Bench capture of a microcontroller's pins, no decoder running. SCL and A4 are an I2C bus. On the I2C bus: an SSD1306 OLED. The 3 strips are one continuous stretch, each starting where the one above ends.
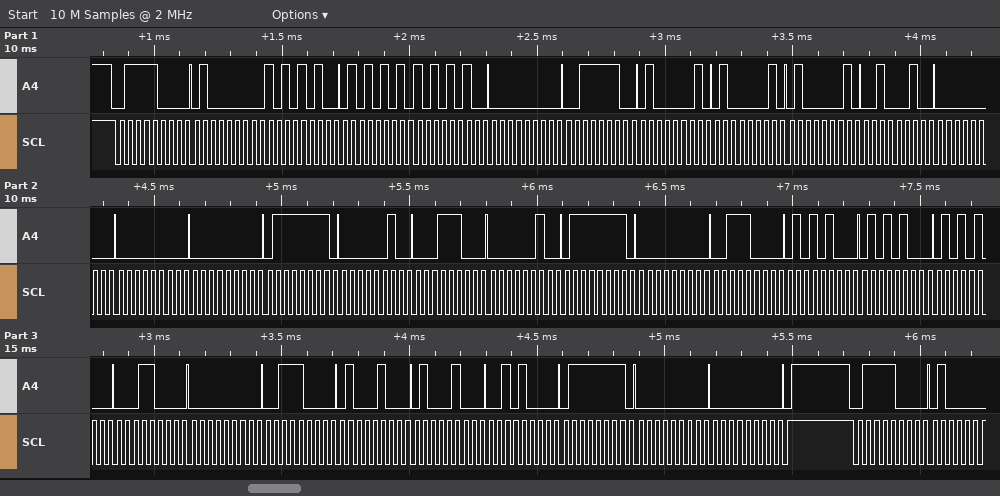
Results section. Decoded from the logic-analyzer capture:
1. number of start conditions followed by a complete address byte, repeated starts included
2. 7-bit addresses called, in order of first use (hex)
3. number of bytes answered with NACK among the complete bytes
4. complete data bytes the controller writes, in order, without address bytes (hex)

2
0x3C
0
40 AA 55 AA 00 3E 41 41 41 22 00 00 00 7F 02 1C 02 7F 00 38 54 54 54 18 00 38 44 44 28 7F 00 00
